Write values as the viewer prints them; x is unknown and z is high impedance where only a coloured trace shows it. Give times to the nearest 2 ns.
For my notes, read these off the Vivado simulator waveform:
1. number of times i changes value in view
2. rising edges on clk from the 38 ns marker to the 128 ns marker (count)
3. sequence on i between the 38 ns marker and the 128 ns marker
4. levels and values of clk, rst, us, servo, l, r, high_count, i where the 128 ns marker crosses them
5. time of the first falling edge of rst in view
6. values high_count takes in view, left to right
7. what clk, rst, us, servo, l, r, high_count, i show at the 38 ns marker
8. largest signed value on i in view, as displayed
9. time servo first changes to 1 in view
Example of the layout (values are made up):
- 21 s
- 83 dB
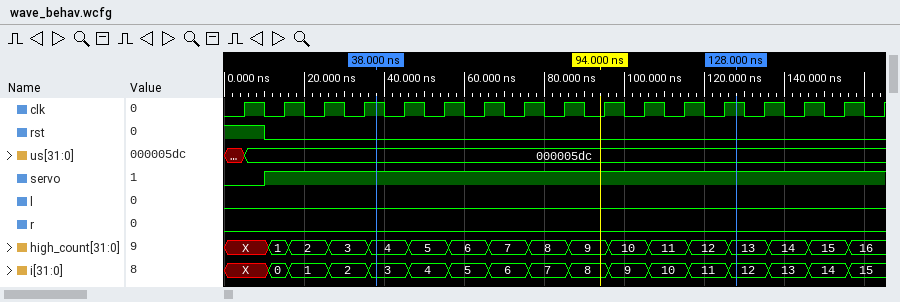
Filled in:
- 16
- 9
- 3, 4, 5, 6, 7, 8, 9, 10, 11, 12
- clk=1, rst=0, us=000005dc, servo=1, l=0, r=0, high_count=13, i=12
- 10 ns
- X, 1, 2, 3, 4, 5, 6, 7, 8, 9, 10, 11, 12, 13, 14, 15, 16
- clk=1, rst=0, us=000005dc, servo=1, l=0, r=0, high_count=4, i=3
- 15
- 10 ns
